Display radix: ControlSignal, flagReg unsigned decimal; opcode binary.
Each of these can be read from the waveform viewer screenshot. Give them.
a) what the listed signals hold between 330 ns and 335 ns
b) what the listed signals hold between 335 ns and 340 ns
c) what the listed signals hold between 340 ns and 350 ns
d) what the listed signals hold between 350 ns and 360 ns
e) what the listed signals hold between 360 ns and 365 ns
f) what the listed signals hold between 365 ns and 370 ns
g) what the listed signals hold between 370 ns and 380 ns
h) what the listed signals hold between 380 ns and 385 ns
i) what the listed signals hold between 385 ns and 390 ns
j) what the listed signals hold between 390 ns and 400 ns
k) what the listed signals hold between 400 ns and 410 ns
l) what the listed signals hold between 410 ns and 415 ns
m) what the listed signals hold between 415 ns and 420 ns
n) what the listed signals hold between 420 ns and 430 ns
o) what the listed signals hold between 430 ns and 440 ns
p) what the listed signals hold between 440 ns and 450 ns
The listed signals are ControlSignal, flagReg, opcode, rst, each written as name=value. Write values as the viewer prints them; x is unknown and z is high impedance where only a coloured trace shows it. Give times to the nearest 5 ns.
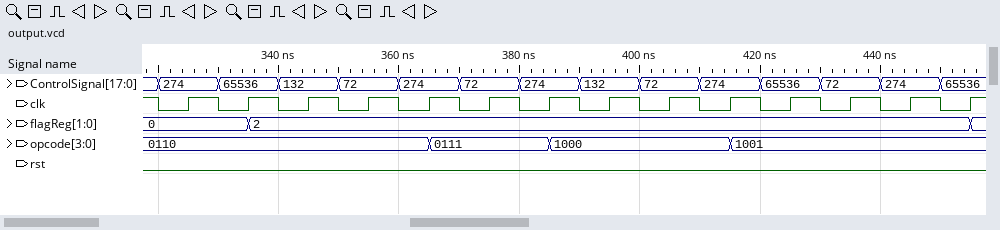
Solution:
ControlSignal=65536, flagReg=0, opcode=0110, rst=0
ControlSignal=65536, flagReg=2, opcode=0110, rst=0
ControlSignal=132, flagReg=2, opcode=0110, rst=0
ControlSignal=72, flagReg=2, opcode=0110, rst=0
ControlSignal=274, flagReg=2, opcode=0110, rst=0
ControlSignal=274, flagReg=2, opcode=0111, rst=0
ControlSignal=72, flagReg=2, opcode=0111, rst=0
ControlSignal=274, flagReg=2, opcode=0111, rst=0
ControlSignal=274, flagReg=2, opcode=1000, rst=0
ControlSignal=132, flagReg=2, opcode=1000, rst=0
ControlSignal=72, flagReg=2, opcode=1000, rst=0
ControlSignal=274, flagReg=2, opcode=1000, rst=0
ControlSignal=274, flagReg=2, opcode=1001, rst=0
ControlSignal=65536, flagReg=2, opcode=1001, rst=0
ControlSignal=72, flagReg=2, opcode=1001, rst=0
ControlSignal=274, flagReg=2, opcode=1001, rst=0
